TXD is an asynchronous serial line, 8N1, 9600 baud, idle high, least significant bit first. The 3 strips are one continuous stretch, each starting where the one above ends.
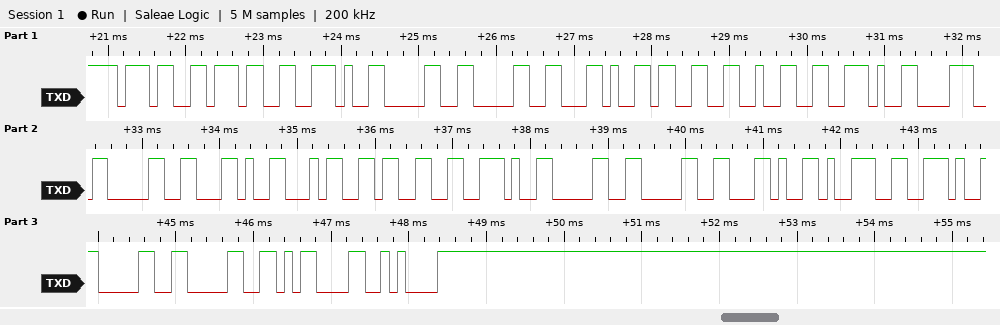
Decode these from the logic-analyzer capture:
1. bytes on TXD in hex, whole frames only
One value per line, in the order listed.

0x37 0x37 0x2E 0x30 0x30 0x2C 0x33 0x32 0x2E 0x38 0x30 0x2C 0x34 0x33 0x2E 0x30 0x30 0x2C 0x39 0x2E 0x30 0x30 0x0D 0x0A
